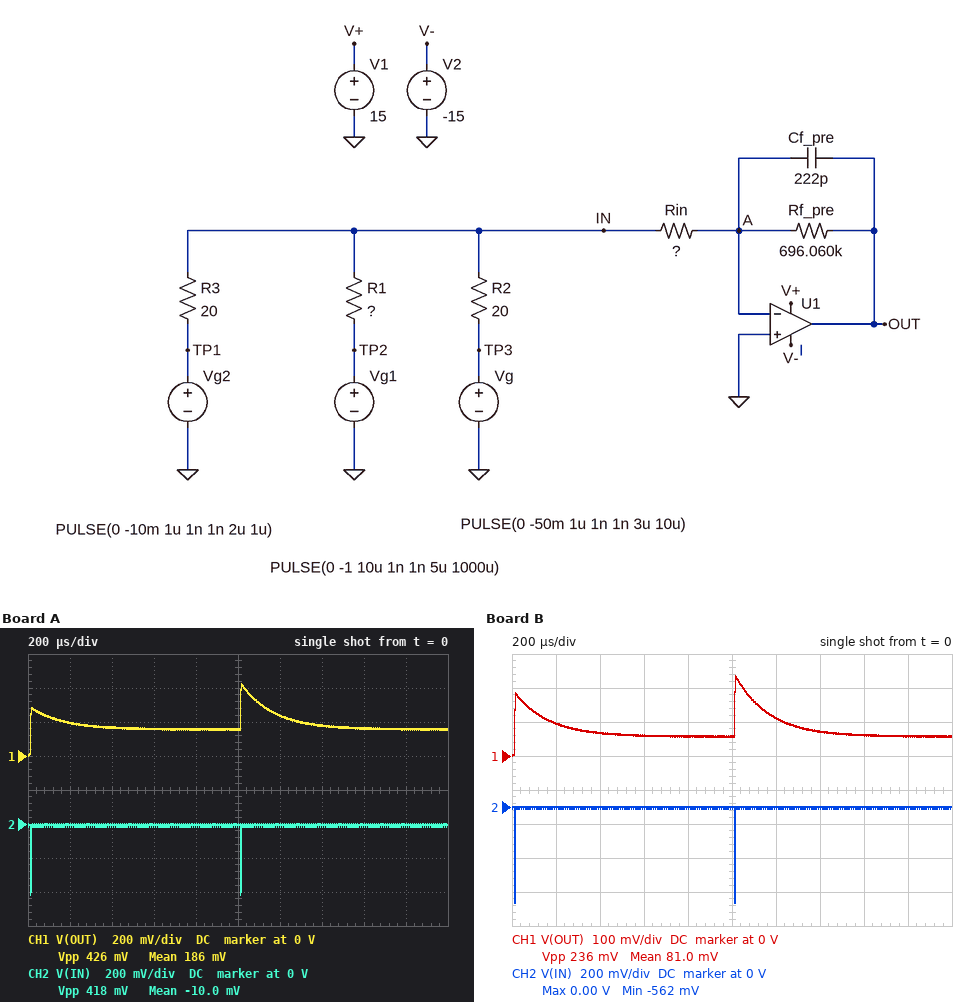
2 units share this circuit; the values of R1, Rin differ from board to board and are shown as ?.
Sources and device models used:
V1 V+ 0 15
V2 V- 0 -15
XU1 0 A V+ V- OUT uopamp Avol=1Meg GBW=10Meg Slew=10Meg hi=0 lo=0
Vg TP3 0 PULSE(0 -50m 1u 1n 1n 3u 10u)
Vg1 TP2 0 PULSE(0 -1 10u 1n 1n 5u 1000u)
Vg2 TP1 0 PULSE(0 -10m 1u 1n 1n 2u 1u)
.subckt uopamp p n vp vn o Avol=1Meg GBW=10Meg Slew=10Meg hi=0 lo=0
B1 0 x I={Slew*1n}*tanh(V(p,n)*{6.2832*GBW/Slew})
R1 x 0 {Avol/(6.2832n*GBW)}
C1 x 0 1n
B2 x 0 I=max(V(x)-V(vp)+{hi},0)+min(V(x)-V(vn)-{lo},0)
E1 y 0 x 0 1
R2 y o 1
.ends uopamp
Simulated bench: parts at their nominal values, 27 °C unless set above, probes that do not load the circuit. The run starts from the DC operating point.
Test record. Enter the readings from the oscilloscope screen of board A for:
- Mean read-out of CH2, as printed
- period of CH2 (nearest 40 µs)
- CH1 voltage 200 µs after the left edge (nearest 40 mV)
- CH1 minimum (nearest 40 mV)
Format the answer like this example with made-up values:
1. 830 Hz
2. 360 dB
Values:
1. -10.0 mV
2. 1.00 ms
3. 200 mV
4. 0 V
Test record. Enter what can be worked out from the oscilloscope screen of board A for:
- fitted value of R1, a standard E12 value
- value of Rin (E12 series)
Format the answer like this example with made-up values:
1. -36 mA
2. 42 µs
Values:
1. 15 Ω
2. 33 kΩ
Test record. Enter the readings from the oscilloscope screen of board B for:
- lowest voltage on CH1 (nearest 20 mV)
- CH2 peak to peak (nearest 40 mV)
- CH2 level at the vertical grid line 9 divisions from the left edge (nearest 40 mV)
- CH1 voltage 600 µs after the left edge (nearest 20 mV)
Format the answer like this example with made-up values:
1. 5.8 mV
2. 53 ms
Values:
1. 0 V
2. 560 mV
3. 0 V
4. 60 mV
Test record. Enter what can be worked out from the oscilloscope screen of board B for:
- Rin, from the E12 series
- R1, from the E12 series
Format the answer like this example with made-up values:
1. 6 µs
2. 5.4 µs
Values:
1. 68 kΩ
2. 8.2 Ω
